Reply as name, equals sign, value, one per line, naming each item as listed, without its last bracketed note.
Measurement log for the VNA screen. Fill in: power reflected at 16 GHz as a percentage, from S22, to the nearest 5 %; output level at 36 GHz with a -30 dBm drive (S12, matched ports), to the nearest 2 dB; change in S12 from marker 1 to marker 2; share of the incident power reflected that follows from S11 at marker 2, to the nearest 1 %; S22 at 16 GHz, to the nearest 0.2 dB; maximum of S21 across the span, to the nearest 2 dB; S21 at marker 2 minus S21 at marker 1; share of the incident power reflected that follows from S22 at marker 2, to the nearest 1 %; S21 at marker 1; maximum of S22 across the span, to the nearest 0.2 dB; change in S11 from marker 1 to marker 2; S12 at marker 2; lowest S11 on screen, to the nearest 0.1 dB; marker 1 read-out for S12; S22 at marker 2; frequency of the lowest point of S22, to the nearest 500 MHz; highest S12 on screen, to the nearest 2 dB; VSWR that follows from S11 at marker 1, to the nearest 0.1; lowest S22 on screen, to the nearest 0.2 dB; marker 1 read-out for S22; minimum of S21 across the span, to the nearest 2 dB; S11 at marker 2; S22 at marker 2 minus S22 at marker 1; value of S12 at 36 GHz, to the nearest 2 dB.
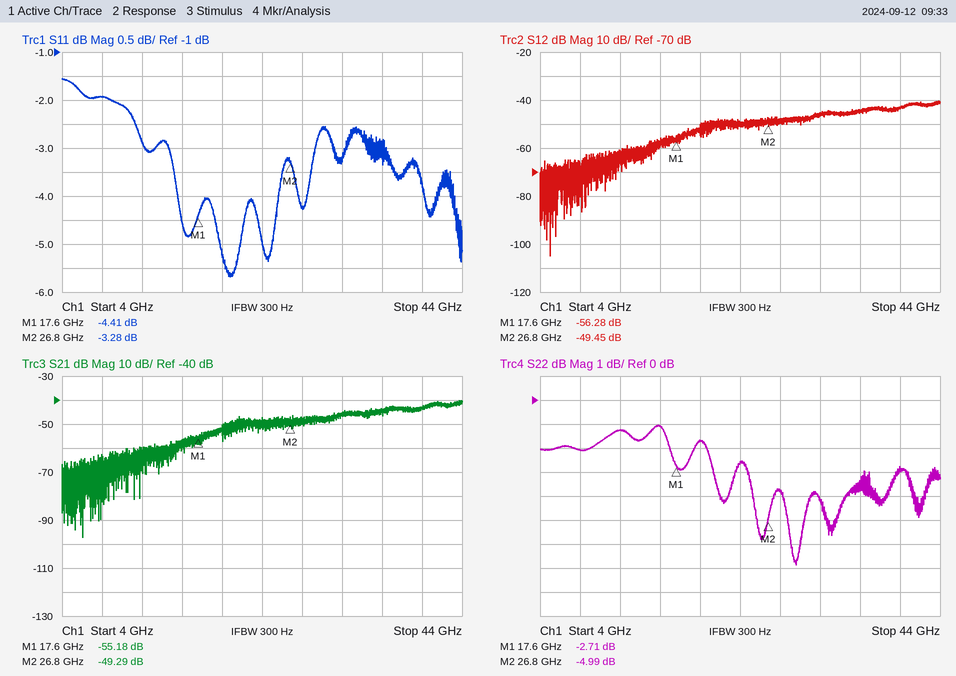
power reflected at 16 GHz as a percentage, from S22, to the nearest 5 % = 80 %
output level at 36 GHz with a -30 dBm drive (S12, matched ports), to the nearest 2 dB = -74 dBm
change in S12 from marker 1 to marker 2 = 6.83 dB
share of the incident power reflected that follows from S11 at marker 2, to the nearest 1 % = 47 %
S22 at 16 GHz, to the nearest 0.2 dB = -1.0 dB
maximum of S21 across the span, to the nearest 2 dB = -40 dB
S21 at marker 2 minus S21 at marker 1 = 5.89 dB
share of the incident power reflected that follows from S22 at marker 2, to the nearest 1 % = 32 %
S21 at marker 1 = -55.18 dB
maximum of S22 across the span, to the nearest 0.2 dB = -1.0 dB
change in S11 from marker 1 to marker 2 = 1.13 dB
S12 at marker 2 = -49.45 dB
lowest S11 on screen, to the nearest 0.1 dB = -5.7 dB
marker 1 read-out for S12 = -56.28 dB
S22 at marker 2 = -4.99 dB
frequency of the lowest point of S22, to the nearest 500 MHz = 29.5 GHz
highest S12 on screen, to the nearest 2 dB = -40 dB
VSWR that follows from S11 at marker 1, to the nearest 0.1 = 4.0
lowest S22 on screen, to the nearest 0.2 dB = -6.8 dB
marker 1 read-out for S22 = -2.71 dB
minimum of S21 across the span, to the nearest 2 dB = -98 dB
S11 at marker 2 = -3.28 dB
S22 at marker 2 minus S22 at marker 1 = -2.28 dB
value of S12 at 36 GHz, to the nearest 2 dB = -44 dB
